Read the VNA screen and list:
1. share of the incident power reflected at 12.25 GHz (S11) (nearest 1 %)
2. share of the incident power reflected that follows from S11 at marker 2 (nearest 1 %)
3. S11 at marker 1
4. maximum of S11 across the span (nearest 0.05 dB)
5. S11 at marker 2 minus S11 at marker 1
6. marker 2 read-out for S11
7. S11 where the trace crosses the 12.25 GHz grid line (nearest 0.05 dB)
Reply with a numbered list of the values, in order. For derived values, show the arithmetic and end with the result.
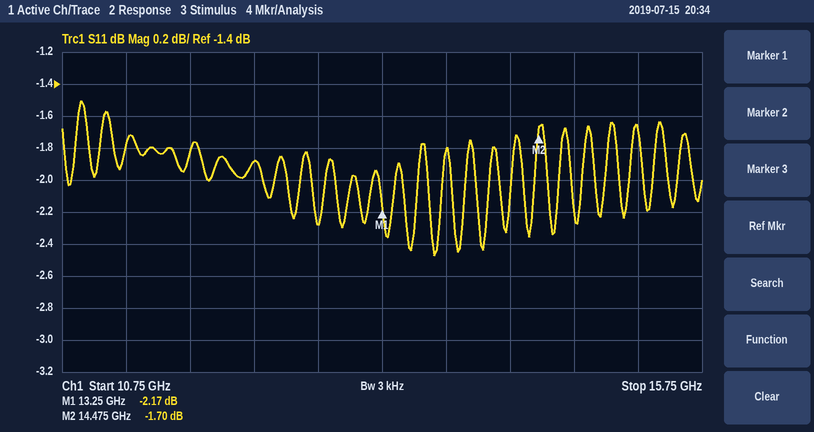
1. 10^(-1.9/10) ≈ 65 %
2. 10^(-1.7/10) ≈ 68 %
3. -2.17 dB
4. -1.50 dB
5. -1.7 − (-2.17) = 0.47 dB
6. -1.70 dB
7. -1.90 dB
